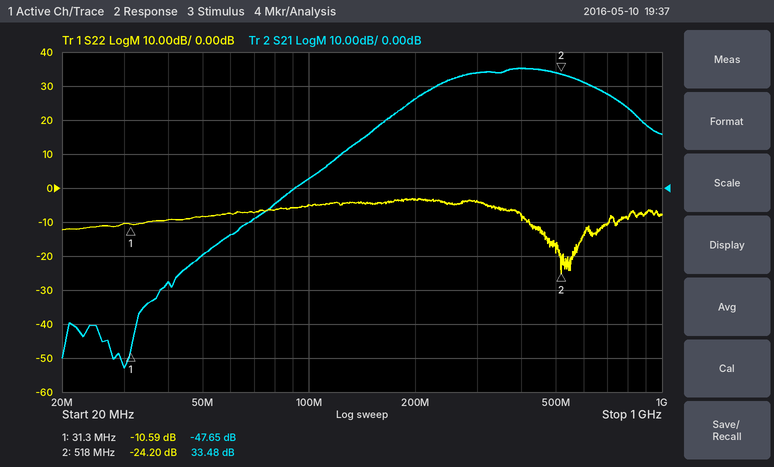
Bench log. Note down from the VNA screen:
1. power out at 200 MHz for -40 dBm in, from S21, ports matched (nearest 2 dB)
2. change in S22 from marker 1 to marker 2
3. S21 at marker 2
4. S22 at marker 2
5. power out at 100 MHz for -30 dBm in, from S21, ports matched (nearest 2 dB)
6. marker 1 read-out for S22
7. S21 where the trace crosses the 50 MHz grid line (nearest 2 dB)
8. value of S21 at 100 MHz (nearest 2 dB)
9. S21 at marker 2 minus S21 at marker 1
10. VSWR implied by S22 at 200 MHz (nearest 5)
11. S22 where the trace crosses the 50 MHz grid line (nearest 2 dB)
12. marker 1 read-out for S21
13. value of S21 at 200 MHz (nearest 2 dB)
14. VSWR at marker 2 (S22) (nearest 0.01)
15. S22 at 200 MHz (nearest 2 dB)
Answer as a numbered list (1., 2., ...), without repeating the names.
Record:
1. -14 dBm
2. -13.61 dB
3. 33.48 dB
4. -24.20 dB
5. -28 dBm
6. -10.59 dB
7. -20 dB
8. 2 dB
9. 81.13 dB
10. 5
11. -8 dB
12. -47.65 dB
13. 26 dB
14. 1.13
15. -4 dB
